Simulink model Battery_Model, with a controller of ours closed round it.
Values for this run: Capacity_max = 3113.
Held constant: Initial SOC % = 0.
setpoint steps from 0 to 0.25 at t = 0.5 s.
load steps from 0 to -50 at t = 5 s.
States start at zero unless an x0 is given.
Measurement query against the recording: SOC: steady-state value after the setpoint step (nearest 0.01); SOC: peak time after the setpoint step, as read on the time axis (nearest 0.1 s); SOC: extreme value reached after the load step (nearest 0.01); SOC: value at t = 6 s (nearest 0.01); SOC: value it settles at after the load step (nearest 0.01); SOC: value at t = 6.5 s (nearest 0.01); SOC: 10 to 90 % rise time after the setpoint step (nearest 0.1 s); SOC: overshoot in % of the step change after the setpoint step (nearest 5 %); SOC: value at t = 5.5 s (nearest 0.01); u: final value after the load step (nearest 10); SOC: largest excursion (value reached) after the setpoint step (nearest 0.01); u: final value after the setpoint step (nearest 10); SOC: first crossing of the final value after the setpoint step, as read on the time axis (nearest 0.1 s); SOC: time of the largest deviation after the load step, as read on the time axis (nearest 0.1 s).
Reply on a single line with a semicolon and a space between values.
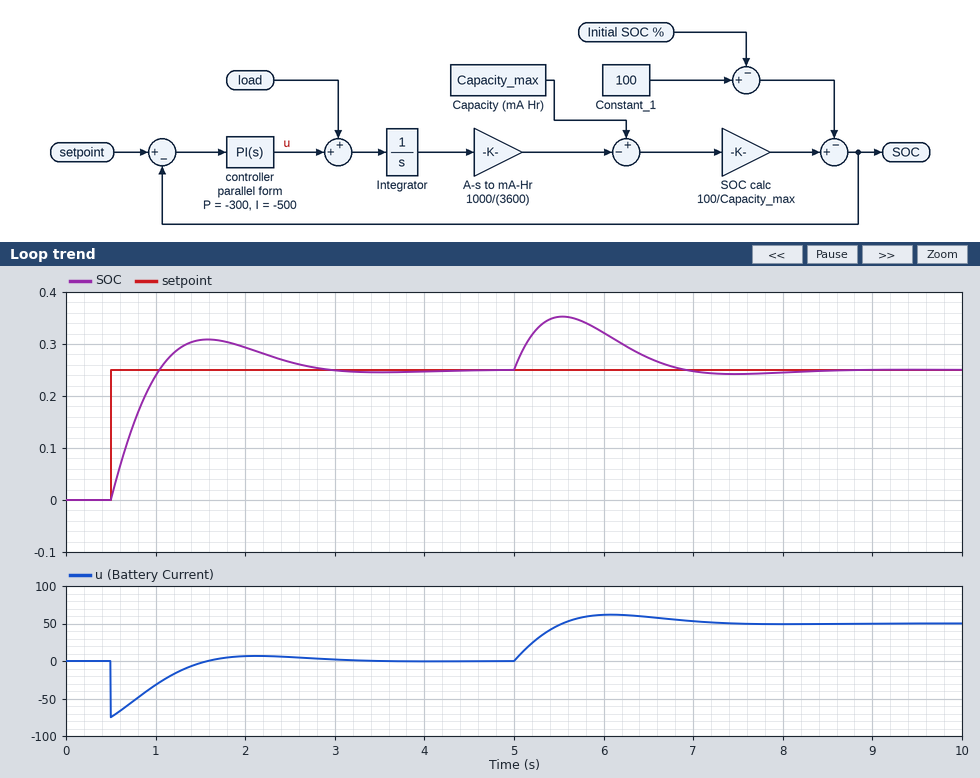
0.25; 1.6 s; 0.35; 0.32; 0.25; 0.27; 0.4 s; 25 %; 0.35; 50; 0.31; 0; 1.0 s; 5.5 s
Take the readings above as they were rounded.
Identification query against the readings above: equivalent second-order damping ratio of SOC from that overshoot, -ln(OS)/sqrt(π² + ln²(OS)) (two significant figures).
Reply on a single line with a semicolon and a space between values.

0.40
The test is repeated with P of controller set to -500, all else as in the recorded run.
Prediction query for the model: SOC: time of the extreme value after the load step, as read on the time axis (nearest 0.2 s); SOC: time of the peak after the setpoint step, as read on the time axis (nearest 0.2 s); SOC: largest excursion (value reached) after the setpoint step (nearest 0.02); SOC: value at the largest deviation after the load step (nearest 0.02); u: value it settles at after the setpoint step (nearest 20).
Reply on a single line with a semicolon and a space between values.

5.4 s; 1.4 s; 0.28; 0.32; 0
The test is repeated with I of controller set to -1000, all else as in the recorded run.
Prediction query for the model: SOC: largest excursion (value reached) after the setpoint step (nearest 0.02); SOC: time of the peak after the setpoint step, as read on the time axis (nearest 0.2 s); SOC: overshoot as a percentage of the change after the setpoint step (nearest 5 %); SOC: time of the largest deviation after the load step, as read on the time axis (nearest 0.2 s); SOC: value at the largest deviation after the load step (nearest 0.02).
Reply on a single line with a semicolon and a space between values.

0.34; 1.4 s; 35 %; 5.4 s; 0.34
